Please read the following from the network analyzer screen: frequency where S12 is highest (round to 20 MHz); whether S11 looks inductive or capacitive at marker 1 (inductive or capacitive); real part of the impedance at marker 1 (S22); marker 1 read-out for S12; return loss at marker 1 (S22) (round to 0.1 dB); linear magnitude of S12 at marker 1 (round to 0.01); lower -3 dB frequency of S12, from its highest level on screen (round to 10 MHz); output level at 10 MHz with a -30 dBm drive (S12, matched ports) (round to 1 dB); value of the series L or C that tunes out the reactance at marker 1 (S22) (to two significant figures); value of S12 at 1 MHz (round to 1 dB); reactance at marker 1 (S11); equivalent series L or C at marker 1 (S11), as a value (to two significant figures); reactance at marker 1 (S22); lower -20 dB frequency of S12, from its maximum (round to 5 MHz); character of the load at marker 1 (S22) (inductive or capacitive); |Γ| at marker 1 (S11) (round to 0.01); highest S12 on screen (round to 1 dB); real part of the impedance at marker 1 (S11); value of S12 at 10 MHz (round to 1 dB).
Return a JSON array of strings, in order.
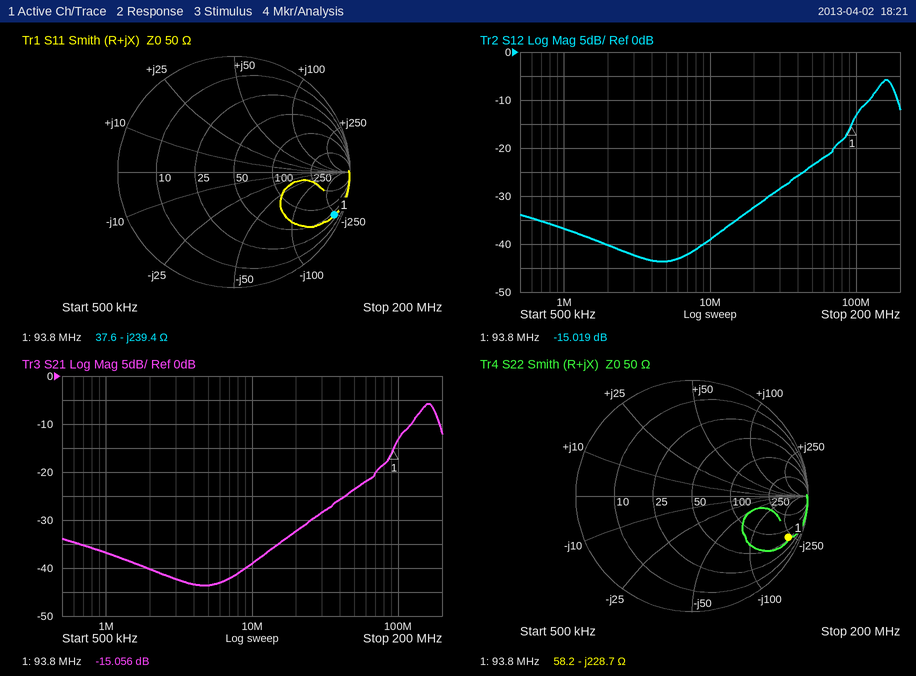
["160 MHz", "capacitive", "58.2 Ω", "-15.019 dB", "0.9 dB", "0.18", "130 MHz", "-69 dBm", "390 nH", "-37 dB", "-239.4 Ω", "7.1 pF", "-228.7 Ω", "40 MHz", "capacitive", "0.94", "-6 dB", "37.6 Ω", "-39 dB"]
